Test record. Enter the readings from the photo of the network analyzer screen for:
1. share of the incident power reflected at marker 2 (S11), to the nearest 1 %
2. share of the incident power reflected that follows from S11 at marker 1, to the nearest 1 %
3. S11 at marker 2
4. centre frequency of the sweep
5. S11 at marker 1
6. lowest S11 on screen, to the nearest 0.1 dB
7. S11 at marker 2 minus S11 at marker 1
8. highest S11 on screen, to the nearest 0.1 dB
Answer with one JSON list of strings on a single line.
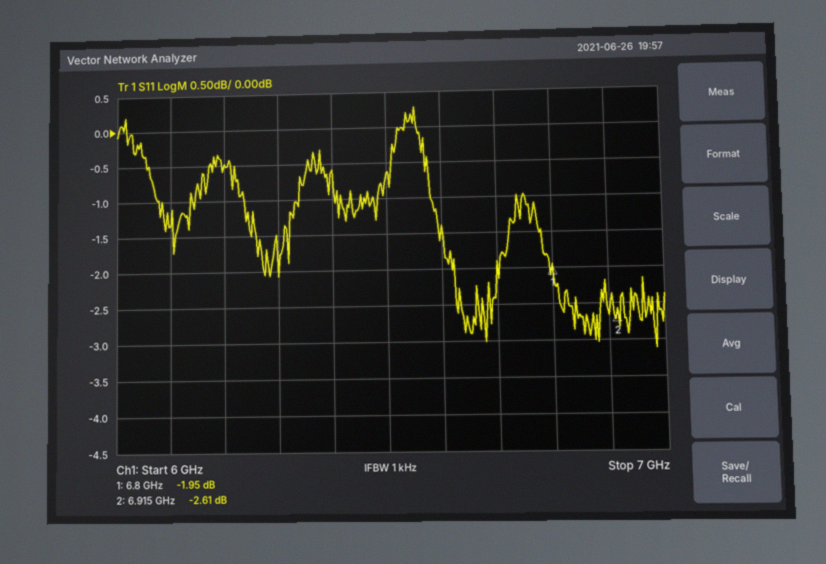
["55 %", "64 %", "-2.61 dB", "6.5 GHz", "-1.95 dB", "-3.1 dB", "-0.66 dB", "0.3 dB"]
